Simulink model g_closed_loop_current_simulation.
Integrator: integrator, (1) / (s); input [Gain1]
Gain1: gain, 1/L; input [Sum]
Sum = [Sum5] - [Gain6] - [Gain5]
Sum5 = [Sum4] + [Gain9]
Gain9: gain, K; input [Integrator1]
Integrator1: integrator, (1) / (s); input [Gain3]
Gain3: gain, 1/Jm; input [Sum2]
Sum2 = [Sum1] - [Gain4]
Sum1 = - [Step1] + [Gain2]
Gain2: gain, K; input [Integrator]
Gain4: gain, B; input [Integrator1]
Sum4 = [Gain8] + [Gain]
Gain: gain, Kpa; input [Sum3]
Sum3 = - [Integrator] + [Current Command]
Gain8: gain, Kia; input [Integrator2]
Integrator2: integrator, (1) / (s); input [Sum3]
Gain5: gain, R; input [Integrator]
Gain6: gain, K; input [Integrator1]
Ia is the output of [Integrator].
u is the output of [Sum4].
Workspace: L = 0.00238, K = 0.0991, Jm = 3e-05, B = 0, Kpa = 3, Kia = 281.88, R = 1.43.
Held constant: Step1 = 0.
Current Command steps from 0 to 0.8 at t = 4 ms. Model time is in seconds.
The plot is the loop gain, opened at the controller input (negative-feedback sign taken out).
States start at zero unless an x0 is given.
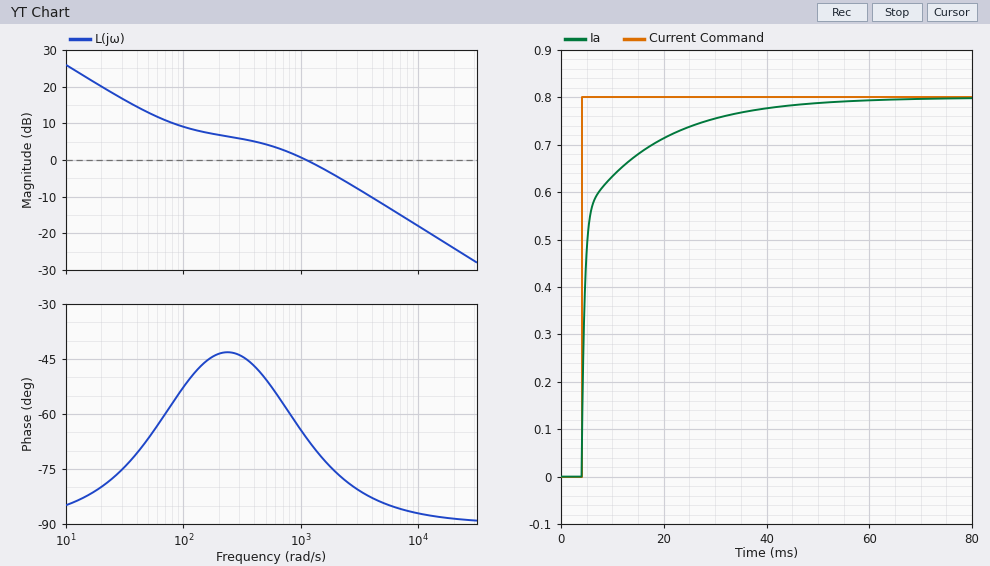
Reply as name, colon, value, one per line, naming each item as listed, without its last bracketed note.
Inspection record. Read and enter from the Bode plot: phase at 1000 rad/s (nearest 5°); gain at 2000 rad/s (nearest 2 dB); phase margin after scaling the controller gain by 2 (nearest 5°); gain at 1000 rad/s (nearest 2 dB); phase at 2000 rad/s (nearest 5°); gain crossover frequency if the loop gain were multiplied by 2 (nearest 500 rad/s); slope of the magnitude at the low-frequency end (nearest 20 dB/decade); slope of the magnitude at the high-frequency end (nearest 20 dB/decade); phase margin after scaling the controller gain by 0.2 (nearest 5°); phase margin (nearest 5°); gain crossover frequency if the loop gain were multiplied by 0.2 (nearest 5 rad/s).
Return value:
phase at 1000 rad/s: -65°
gain at 2000 rad/s: -4 dB
phase margin after scaling the controller gain by 2: 100°
gain at 1000 rad/s: 0 dB
phase at 2000 rad/s: -75°
gain crossover frequency if the loop gain were multiplied by 2: 2500 rad/s
slope of the magnitude at the low-frequency end: -20 dB/decade
slope of the magnitude at the high-frequency end: -20 dB/decade
phase margin after scaling the controller gain by 0.2: 110°
phase margin: 115°
gain crossover frequency if the loop gain were multiplied by 0.2: 45 rad/s
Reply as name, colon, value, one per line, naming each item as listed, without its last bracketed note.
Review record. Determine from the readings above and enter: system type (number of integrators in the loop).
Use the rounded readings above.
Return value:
system type: 1
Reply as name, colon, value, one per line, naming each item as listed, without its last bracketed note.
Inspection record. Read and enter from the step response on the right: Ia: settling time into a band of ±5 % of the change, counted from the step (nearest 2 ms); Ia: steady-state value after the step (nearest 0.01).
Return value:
Ia: settling time into a band of ±5 % of the change, counted from the step: 28 ms
Ia: steady-state value after the step: 0.80
